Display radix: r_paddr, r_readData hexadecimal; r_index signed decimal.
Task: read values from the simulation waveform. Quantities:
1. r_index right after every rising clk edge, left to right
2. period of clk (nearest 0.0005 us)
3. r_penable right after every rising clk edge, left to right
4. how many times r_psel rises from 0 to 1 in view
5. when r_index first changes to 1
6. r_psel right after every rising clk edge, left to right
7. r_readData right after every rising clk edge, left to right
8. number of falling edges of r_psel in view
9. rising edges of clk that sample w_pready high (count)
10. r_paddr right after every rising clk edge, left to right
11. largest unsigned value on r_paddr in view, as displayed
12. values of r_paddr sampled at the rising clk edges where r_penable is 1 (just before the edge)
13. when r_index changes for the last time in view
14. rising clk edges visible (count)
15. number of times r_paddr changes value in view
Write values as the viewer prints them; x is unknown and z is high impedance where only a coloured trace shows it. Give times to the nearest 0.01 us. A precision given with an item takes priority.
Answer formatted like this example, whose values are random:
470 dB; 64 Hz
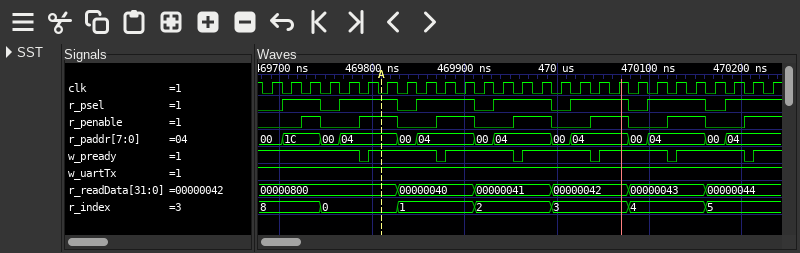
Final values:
8, 8, 8, 0, 0, 0, 0, 1, 1, 1, 1, 2, 2, 2, 2, 3, 3, 3, 3, 4, 4, 4, 4, 5, 5, 5, 5; 0.021 us; 0 0 1 0 0 1 1 0 0 1 1 0 0 1 1 0 0 1 1 0 0 1 1 0 0 1 1; 7; 469.83 us; 0 1 1 0 1 1 1 0 1 1 1 0 1 1 1 0 1 1 1 0 1 1 1 0 1 1 1; 00000800, 00000800, 00000800, 00000800, 00000800, 00000800, 00000800, 00000040, 00000040, 00000040, 00000040, 00000041, 00000041, 00000041, 00000041, 00000042, 00000042, 00000042, 00000042, 00000043, 00000043, 00000043, 00000043, 00000044, 00000044, 00000044, 00000044; 6; 21; 00, 1C, 1C, 00, 04, 04, 04, 00, 04, 04, 04, 00, 04, 04, 04, 00, 04, 04, 04, 00, 04, 04, 04, 00, 04, 04, 04; 1C; 1C, 04, 04, 04, 04, 04, 04, 04, 04, 04, 04, 04, 04; 470.16 us; 27; 13
